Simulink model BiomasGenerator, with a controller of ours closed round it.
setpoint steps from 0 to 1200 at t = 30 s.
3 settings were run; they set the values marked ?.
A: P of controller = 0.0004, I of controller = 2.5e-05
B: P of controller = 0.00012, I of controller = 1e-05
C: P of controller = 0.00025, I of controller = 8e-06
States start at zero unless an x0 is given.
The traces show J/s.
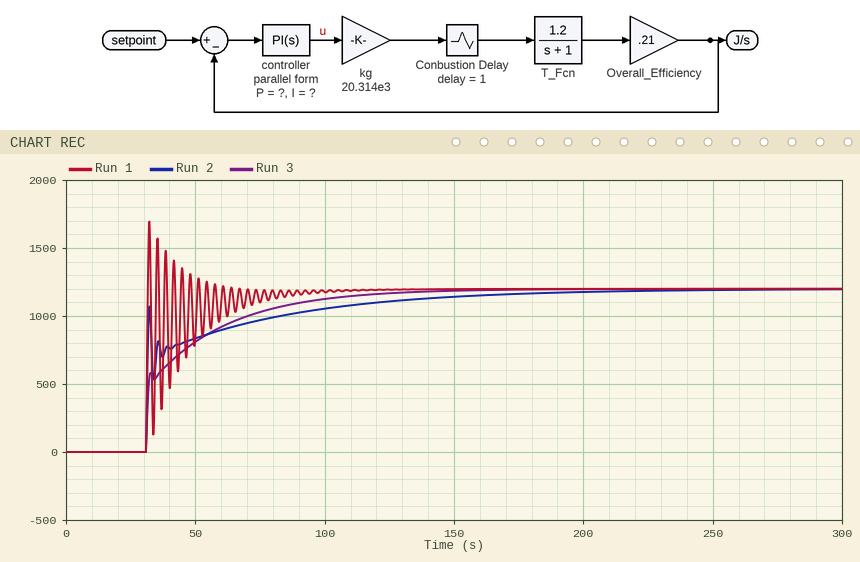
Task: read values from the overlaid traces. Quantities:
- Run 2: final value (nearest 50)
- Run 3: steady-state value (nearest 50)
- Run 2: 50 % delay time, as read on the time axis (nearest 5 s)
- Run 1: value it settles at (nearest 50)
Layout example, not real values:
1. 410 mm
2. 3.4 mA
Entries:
1. 1200
2. 1200
3. 30 s
4. 1200
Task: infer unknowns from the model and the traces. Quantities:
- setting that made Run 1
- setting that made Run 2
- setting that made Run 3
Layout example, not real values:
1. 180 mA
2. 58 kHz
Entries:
1. A
2. C
3. B
